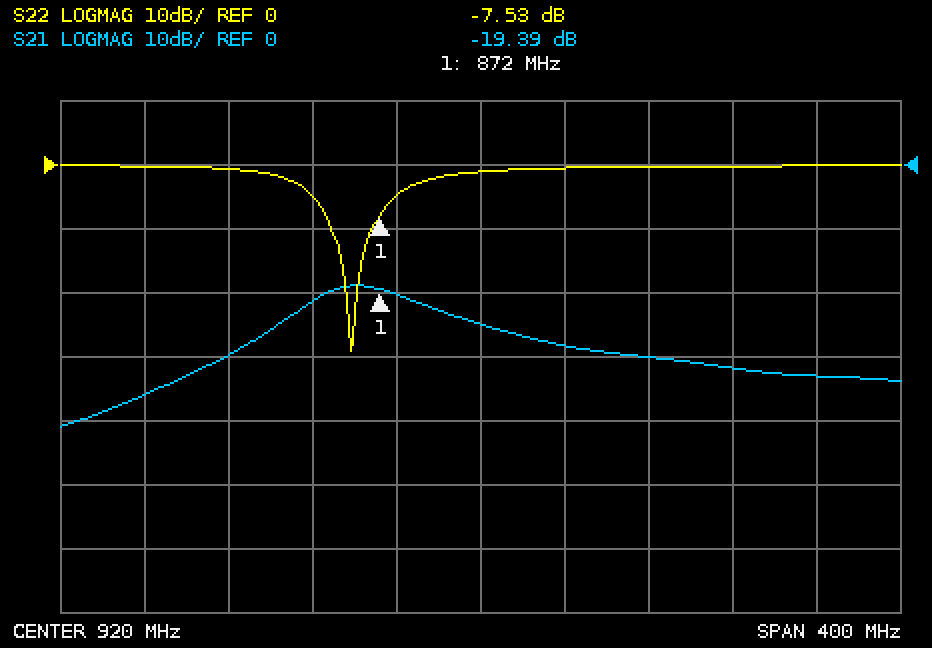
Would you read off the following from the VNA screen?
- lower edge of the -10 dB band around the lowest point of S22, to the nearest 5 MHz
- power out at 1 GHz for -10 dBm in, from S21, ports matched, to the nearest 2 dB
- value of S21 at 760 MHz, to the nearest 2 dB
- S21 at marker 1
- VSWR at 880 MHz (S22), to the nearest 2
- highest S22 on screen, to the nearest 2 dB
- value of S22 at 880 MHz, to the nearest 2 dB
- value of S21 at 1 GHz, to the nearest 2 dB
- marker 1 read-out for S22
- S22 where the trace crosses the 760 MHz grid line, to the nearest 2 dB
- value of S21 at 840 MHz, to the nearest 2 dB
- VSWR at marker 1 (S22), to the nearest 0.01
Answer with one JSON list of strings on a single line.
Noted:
["850 MHz", "-40 dBm", "-36 dB", "-19.39 dB", "4", "0 dB", "-4 dB", "-30 dB", "-7.53 dB", "0 dB", "-22 dB", "2.45"]
